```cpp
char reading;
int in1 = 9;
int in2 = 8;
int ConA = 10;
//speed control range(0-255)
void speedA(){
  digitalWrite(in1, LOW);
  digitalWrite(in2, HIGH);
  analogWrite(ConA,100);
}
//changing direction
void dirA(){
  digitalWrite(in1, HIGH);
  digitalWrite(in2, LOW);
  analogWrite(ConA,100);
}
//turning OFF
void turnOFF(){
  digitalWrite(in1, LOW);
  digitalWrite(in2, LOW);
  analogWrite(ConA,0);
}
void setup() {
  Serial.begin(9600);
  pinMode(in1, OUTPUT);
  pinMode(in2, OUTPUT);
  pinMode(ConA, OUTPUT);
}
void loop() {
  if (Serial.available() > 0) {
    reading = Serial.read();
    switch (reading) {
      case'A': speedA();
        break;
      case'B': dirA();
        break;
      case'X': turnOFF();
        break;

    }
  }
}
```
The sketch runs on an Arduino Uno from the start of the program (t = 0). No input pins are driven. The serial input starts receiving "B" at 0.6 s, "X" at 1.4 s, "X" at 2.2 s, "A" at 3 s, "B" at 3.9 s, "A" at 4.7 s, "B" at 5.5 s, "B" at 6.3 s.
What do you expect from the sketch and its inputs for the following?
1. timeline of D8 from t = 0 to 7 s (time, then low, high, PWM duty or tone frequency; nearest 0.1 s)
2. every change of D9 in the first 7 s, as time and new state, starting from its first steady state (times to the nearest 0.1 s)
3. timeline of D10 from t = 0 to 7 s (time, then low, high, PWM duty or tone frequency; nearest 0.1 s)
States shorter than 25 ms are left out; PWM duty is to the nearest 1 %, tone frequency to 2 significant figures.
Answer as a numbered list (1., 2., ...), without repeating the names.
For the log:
1. 0 s low; 3 s high; 3.9 s low; 4.7 s high; 5.5 s low
2. 0 s low; 0.6 s high; 1.4 s low; 3.9 s high; 4.7 s low; 5.5 s high
3. 0 s low; 0.6 s PWM 39 %; 1.4 s low; 3 s PWM 39 %
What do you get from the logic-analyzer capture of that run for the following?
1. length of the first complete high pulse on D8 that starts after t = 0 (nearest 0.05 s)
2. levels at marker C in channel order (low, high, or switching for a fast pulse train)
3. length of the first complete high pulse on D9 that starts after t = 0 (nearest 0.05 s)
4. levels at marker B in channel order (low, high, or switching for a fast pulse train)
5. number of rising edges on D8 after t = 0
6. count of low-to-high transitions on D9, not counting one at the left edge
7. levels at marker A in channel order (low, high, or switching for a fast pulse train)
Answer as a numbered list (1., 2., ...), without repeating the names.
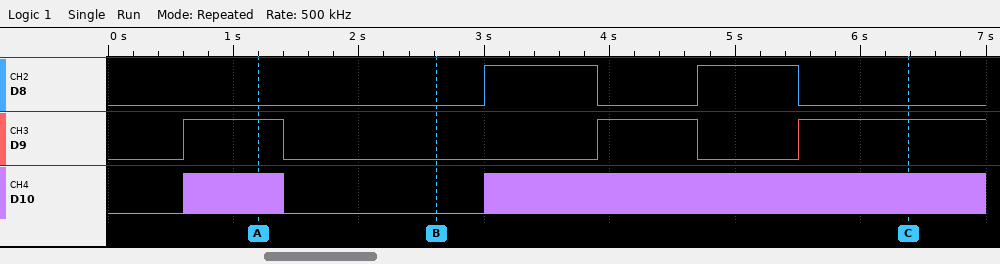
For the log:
1. 0.90 s
2. D8 low, D9 high, D10 switching
3. 0.80 s
4. D8 low, D9 low, D10 low
5. 2
6. 3
7. D8 low, D9 high, D10 switching
